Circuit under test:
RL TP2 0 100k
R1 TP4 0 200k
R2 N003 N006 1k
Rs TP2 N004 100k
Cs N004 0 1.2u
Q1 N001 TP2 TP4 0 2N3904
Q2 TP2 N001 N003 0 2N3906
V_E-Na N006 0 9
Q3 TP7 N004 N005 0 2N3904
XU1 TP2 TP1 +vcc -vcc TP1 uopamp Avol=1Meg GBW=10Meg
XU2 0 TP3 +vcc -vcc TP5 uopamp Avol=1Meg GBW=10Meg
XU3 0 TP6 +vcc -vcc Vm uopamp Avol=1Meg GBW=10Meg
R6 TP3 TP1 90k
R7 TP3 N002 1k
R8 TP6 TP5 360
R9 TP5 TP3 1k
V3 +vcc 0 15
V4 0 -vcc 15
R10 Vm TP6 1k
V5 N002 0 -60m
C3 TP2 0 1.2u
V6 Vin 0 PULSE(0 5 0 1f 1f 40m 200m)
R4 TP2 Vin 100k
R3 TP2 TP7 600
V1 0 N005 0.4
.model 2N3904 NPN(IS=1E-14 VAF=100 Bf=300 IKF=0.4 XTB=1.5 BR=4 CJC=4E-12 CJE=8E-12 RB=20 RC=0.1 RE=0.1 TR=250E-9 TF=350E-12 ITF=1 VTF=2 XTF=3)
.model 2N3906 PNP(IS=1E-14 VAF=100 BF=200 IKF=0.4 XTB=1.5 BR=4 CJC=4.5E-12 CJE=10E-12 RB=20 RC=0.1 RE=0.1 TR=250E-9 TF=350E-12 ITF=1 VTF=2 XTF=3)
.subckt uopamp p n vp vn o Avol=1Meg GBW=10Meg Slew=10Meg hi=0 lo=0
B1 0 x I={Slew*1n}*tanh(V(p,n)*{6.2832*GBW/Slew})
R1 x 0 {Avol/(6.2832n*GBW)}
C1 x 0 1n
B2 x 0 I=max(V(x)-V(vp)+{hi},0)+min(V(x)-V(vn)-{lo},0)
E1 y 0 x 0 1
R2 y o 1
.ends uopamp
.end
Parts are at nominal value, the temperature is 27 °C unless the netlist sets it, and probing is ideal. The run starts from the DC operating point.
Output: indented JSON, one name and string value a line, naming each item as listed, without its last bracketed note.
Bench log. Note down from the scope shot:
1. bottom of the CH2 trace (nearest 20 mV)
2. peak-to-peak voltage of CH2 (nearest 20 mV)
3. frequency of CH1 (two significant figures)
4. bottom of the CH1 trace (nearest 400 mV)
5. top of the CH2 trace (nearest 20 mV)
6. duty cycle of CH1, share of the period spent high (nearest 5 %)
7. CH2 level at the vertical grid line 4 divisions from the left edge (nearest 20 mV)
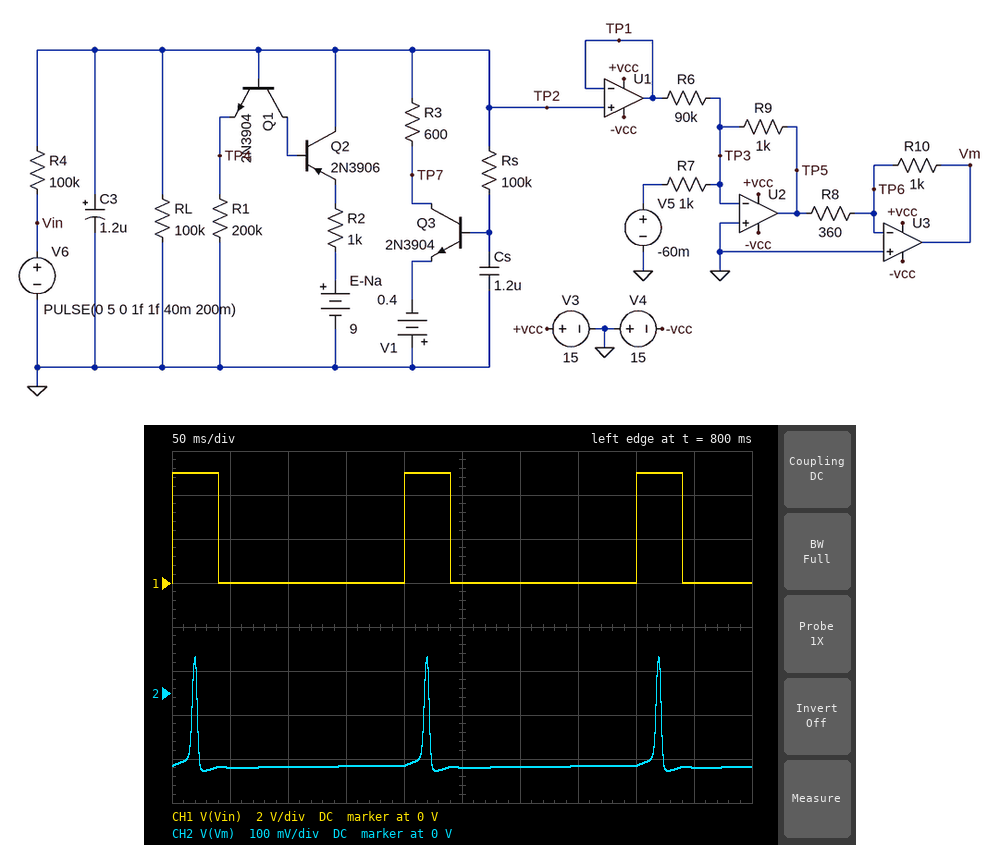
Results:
{
  "bottom of the CH2 trace": "-180 mV",
  "peak-to-peak voltage of CH2": "260 mV",
  "frequency of CH1": "5.0 Hz",
  "bottom of the CH1 trace": "0 V",
  "top of the CH2 trace": "80 mV",
  "duty cycle of CH1, share of the period spent high": "20 %",
  "CH2 level at the vertical grid line 4 divisions from the left edge": "-160 mV"
}
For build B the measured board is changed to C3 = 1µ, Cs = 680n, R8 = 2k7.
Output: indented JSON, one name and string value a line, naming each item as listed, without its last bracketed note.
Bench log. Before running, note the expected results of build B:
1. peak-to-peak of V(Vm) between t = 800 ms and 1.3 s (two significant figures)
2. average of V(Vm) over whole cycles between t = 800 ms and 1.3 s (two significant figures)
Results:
{
  "peak-to-peak of V(Vm) between t = 800 ms and 1.3 s": "32 mV",
  "average of V(Vm) over whole cycles between t = 800 ms and 1.3 s": "-22 mV"
}
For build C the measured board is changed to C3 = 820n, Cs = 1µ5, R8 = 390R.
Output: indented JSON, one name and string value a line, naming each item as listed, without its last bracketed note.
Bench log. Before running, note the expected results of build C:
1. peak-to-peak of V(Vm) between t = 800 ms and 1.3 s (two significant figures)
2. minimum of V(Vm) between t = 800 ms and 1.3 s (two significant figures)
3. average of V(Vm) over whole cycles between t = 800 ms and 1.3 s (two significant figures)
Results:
{
  "peak-to-peak of V(Vm) between t = 800 ms and 1.3 s": "250 mV",
  "minimum of V(Vm) between t = 800 ms and 1.3 s": "-160 mV",
  "average of V(Vm) over whole cycles between t = 800 ms and 1.3 s": "-150 mV"
}
